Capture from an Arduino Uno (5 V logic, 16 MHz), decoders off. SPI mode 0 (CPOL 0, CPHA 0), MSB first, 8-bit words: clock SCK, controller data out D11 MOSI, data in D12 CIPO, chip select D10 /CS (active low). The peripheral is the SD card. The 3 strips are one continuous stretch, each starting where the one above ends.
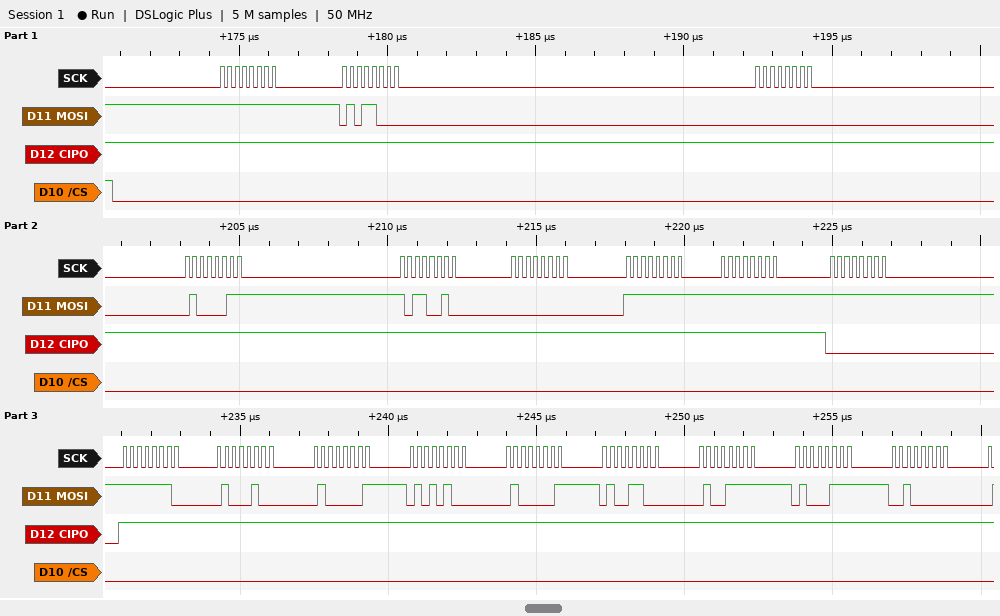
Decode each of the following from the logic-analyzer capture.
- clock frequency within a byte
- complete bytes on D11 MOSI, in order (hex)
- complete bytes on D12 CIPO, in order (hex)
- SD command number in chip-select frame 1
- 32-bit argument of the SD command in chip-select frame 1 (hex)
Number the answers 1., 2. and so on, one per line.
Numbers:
1. 4 MHz
2. 0xFF 0x58 0x00 0x43 0xB2 0x00 0xFF 0xFF 0xFF 0xFE 0x44 0x41 0x54 0x41 0x4C 0x4F 0x47 0x20
3. 0xFF 0xFF 0xFF 0xFF 0xFF 0xFF 0xFF 0xFF 0x00 0xFF 0xFF 0xFF 0xFF 0xFF 0xFF 0xFF 0xFF 0xFF
4. CMD24
5. 0x0043B200
